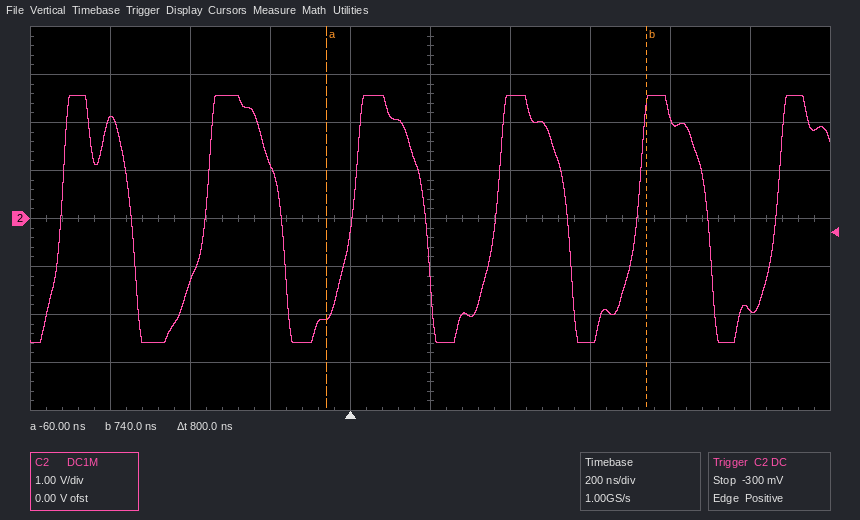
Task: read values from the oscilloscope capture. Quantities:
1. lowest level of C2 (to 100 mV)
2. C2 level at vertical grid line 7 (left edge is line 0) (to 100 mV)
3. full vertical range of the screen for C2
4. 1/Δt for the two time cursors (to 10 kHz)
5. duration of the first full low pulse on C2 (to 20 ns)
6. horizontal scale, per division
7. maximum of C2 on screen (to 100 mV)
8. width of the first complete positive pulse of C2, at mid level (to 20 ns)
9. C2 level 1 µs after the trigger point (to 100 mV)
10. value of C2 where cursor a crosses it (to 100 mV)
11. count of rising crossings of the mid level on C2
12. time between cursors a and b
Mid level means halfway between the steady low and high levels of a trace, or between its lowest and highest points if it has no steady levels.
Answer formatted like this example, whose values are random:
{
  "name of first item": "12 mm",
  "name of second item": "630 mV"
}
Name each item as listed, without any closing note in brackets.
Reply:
{
  "lowest level of C2": "-2.6 V",
  "C2 level at vertical grid line 7 (left edge is line 0)": "-2.6 V",
  "full vertical range of the screen for C2": "8 V",
  "1/Δt for the two time cursors": "1.25 MHz",
  "duration of the first full low pulse on C2": "180 ns",
  "horizontal scale, per division": "200 ns",
  "maximum of C2 on screen": "2.6 V",
  "width of the first complete positive pulse of C2, at mid level": "180 ns",
  "C2 level 1 µs after the trigger point": "-1.9 V",
  "value of C2 where cursor a crosses it": "-2.1 V",
  "count of rising crossings of the mid level on C2": "6",
  "time between cursors a and b": "800 ns"
}
